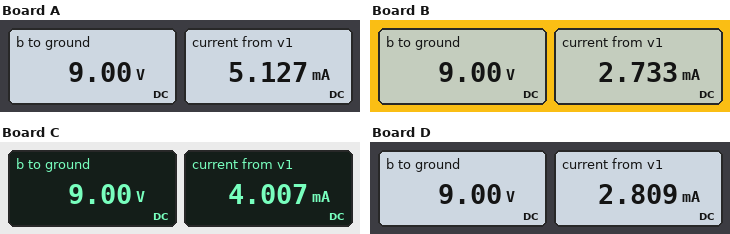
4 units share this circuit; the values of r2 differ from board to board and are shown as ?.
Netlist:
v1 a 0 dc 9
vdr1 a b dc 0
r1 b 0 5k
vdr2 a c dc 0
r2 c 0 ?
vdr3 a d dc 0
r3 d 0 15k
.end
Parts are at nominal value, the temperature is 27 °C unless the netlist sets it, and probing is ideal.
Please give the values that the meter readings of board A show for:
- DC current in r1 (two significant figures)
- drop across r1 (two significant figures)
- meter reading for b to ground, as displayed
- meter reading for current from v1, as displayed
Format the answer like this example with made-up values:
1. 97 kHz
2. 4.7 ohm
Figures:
1. 1.8 mA
2. 9.0 V
3. 9.00 V
4. 5.127 mA
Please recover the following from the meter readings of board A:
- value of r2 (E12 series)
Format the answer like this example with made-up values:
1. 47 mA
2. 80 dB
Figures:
1. 3.3 kΩ
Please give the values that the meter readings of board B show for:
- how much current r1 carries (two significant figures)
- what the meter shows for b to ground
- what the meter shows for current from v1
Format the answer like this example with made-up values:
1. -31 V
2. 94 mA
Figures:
1. 1.8 mA
2. 9.00 V
3. 2.733 mA
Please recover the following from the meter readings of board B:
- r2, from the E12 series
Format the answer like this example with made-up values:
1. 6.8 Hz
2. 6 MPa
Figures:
1. 27 kΩ
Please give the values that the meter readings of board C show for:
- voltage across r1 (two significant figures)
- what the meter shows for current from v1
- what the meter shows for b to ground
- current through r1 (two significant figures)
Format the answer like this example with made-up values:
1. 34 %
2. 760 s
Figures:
1. 9.0 V
2. 4.007 mA
3. 9.00 V
4. 1.8 mA
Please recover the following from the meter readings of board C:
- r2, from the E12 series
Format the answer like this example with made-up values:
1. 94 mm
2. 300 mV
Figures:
1. 5.6 kΩ
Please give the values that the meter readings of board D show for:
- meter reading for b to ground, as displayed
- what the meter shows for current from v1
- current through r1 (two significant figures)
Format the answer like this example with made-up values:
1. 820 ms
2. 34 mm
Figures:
1. 9.00 V
2. 2.809 mA
3. 1.8 mA
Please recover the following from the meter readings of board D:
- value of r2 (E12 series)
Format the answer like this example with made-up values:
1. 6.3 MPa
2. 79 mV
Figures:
1. 22 kΩ
